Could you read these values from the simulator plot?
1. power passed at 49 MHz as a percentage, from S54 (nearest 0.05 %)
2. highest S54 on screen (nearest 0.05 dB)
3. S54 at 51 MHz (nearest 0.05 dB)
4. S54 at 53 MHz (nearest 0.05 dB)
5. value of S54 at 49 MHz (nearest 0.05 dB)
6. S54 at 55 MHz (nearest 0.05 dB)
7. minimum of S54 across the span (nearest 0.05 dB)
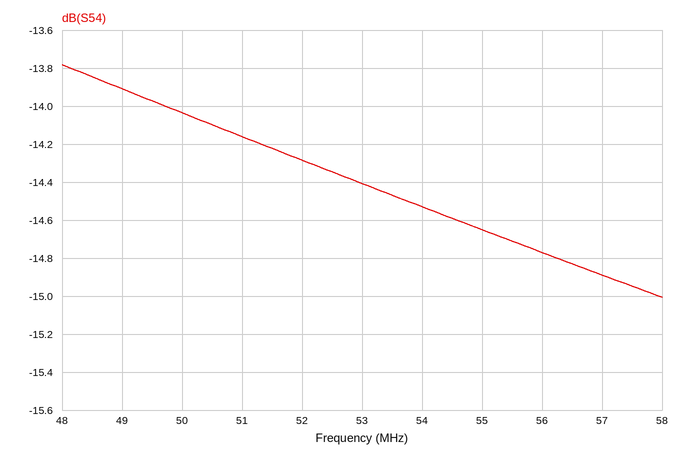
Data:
4.05 %
-13.80 dB
-14.15 dB
-14.40 dB
-13.90 dB
-14.65 dB
-15.00 dB
